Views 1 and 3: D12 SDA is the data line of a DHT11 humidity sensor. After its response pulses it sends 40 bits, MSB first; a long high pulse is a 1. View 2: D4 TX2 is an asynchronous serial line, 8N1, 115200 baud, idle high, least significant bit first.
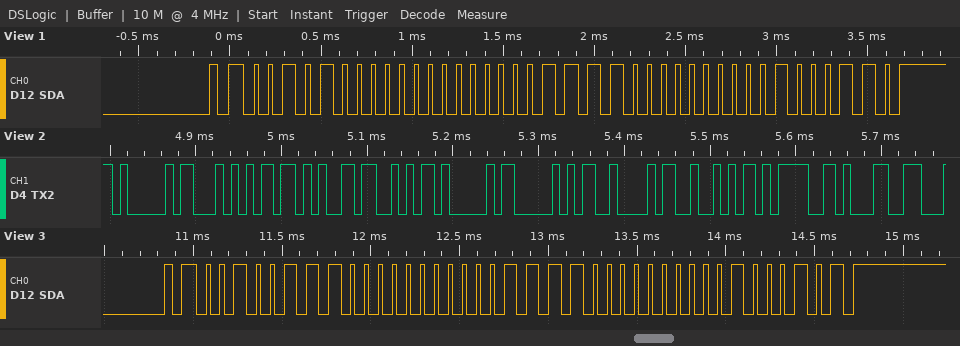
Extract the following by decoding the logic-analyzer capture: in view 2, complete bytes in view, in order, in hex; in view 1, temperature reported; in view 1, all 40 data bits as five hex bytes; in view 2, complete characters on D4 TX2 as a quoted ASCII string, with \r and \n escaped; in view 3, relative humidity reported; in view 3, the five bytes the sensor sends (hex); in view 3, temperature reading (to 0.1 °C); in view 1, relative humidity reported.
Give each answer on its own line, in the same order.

0x41 0x54 0x2B 0x53 0x41 0x50 0x42 0x52 0x3D 0x31
30.0 °C
28 00 1E 00 46
"AT+SAPBR=1"
39 %
27 00 1E 00 45
30.0 °C
40 %
